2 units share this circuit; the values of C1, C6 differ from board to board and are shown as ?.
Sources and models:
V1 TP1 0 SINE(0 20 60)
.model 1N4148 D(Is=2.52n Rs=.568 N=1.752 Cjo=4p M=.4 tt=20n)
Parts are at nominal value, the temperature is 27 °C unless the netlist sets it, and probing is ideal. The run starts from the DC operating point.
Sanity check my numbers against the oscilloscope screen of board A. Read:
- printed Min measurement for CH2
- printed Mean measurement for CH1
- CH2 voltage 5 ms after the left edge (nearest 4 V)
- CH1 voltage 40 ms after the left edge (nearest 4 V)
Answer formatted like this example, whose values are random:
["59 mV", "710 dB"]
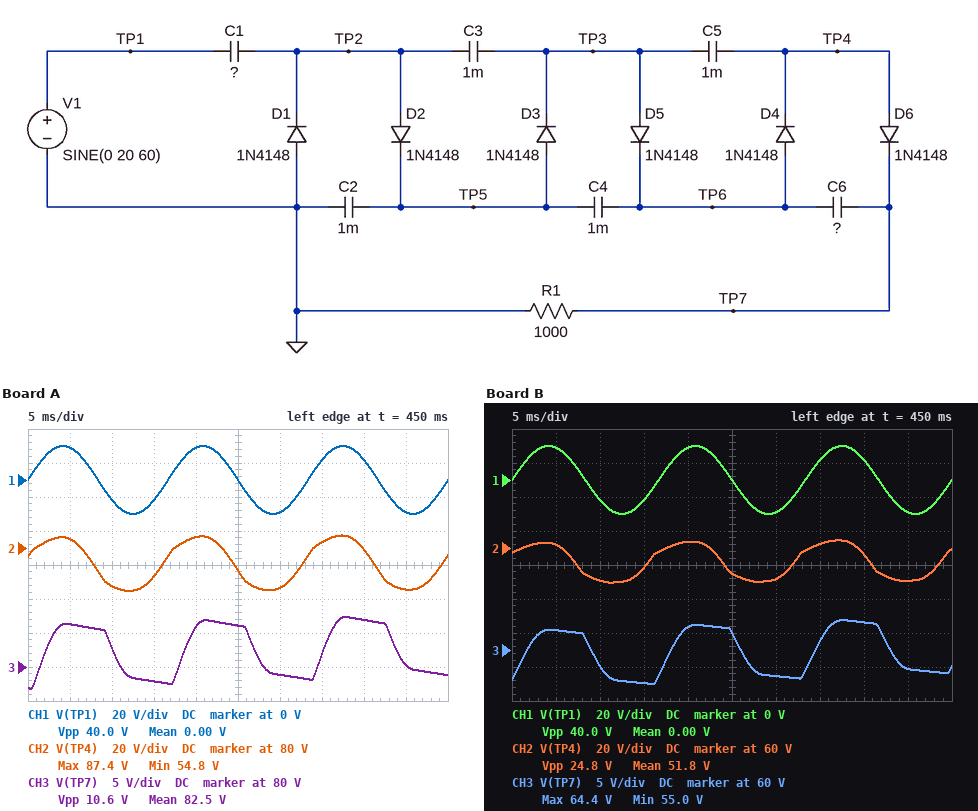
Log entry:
["54.8 V", "0.00 V", "84 V", "12 V"]
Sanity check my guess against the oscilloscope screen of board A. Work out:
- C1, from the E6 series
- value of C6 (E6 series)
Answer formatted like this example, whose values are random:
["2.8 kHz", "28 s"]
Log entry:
["2.2 mF", "2.2 mF"]
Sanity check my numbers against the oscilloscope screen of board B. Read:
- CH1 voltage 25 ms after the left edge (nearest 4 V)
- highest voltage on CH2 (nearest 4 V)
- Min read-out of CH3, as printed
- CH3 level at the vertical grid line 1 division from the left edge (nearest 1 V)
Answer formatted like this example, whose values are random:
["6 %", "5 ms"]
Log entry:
["0 V", "64 V", "55.0 V", "63 V"]
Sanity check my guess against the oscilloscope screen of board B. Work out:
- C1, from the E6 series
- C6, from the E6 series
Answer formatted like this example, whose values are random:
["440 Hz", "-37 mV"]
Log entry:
["470 µF", "3.3 mF"]
